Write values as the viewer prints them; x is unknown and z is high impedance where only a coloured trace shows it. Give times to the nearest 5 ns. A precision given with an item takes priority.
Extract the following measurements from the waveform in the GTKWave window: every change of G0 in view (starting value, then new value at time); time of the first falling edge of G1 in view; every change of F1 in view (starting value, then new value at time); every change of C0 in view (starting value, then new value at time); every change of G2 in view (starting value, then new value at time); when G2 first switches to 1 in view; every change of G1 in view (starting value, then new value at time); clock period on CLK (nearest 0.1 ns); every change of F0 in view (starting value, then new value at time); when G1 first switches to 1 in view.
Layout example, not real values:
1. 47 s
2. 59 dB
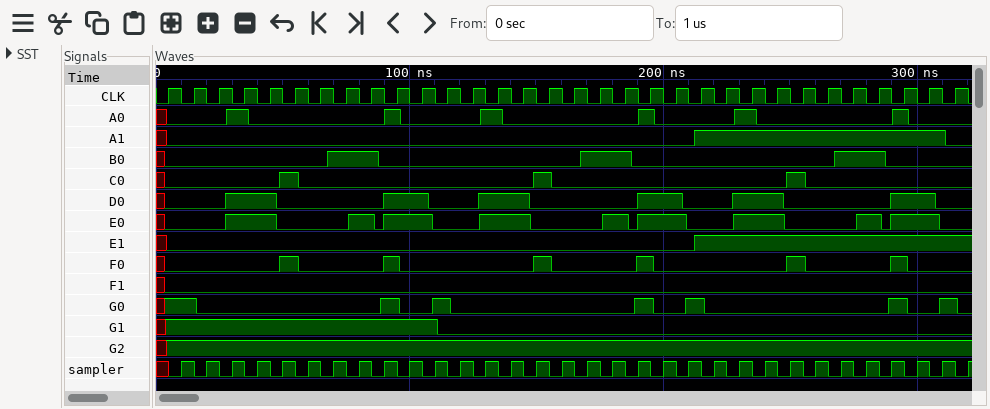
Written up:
1. x, 1 at 5 ns, 0 at 15 ns, 1 at 90 ns, 0 at 95 ns, 1 at 110 ns, 0 at 115 ns, 1 at 190 ns, 0 at 195 ns, 1 at 210 ns, 0 at 215 ns, 1 at 290 ns, 0 at 295 ns, 1 at 310 ns, 0 at 315 ns
2. 110 ns
3. x, 0 at 5 ns
4. x, 0 at 5 ns, 1 at 50 ns, 0 at 55 ns, 1 at 150 ns, 0 at 155 ns, 1 at 250 ns, 0 at 255 ns
5. x, 1 at 5 ns
6. 5 ns
7. x, 1 at 5 ns, 0 at 110 ns
8. 10 ns
9. x, 0 at 5 ns, 1 at 50 ns, 0 at 55 ns, 1 at 90 ns, 0 at 95 ns, 1 at 150 ns, 0 at 155 ns, 1 at 190 ns, 0 at 195 ns, 1 at 250 ns, 0 at 255 ns, 1 at 290 ns, 0 at 295 ns
10. 5 ns
